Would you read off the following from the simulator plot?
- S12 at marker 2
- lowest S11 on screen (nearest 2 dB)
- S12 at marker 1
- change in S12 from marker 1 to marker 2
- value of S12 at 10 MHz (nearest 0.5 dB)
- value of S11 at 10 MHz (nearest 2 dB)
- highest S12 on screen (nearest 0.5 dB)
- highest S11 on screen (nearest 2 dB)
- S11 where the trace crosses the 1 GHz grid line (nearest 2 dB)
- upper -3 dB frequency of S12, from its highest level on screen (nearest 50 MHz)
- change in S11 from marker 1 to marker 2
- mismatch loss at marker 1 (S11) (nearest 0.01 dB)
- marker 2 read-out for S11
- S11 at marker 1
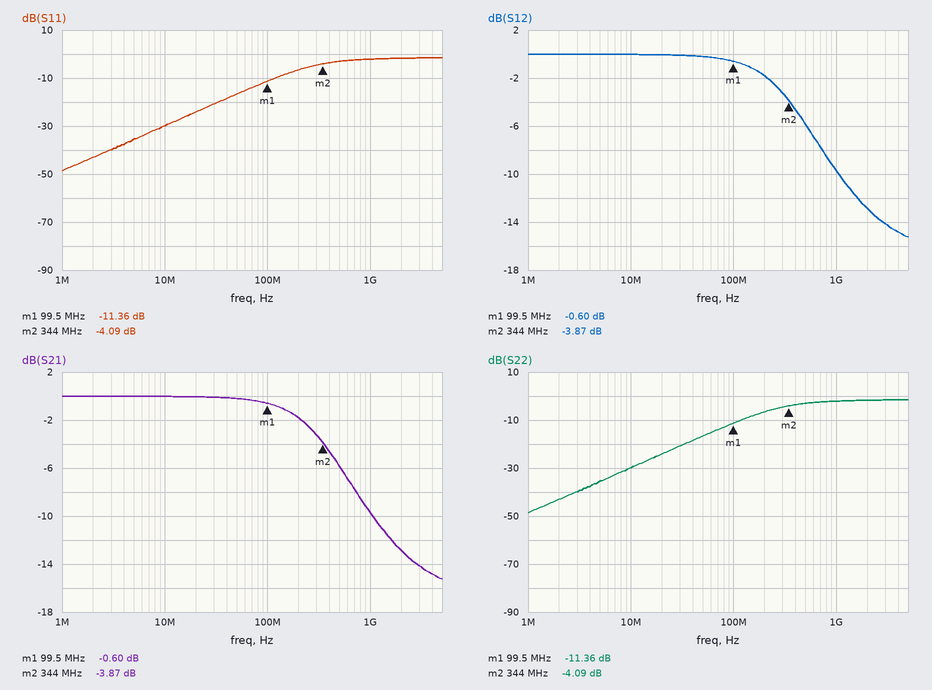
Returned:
-3.87 dB
-48 dB
-0.60 dB
-3.27 dB
0.0 dB
-30 dB
0.0 dB
-2 dB
-2 dB
300 MHz
7.27 dB
0.33 dB
-4.09 dB
-11.36 dB
